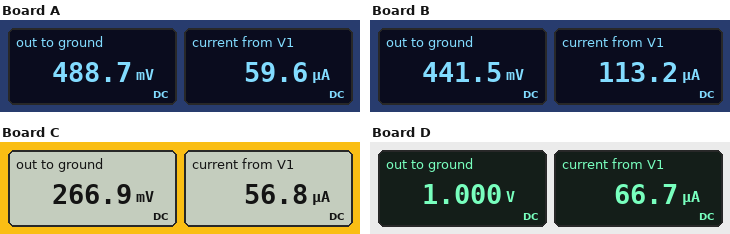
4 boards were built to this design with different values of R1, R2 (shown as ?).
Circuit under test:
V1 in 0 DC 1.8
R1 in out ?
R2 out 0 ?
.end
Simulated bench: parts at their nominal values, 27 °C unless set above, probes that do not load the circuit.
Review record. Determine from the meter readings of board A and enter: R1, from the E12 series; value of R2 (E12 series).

22 kΩ
8.2 kΩ
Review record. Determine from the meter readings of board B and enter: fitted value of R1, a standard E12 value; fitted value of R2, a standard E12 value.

12 kΩ
3.9 kΩ
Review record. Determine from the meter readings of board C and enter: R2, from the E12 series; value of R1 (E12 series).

4.7 kΩ
27 kΩ
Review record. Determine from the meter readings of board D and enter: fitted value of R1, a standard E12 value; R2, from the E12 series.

12 kΩ
15 kΩ
